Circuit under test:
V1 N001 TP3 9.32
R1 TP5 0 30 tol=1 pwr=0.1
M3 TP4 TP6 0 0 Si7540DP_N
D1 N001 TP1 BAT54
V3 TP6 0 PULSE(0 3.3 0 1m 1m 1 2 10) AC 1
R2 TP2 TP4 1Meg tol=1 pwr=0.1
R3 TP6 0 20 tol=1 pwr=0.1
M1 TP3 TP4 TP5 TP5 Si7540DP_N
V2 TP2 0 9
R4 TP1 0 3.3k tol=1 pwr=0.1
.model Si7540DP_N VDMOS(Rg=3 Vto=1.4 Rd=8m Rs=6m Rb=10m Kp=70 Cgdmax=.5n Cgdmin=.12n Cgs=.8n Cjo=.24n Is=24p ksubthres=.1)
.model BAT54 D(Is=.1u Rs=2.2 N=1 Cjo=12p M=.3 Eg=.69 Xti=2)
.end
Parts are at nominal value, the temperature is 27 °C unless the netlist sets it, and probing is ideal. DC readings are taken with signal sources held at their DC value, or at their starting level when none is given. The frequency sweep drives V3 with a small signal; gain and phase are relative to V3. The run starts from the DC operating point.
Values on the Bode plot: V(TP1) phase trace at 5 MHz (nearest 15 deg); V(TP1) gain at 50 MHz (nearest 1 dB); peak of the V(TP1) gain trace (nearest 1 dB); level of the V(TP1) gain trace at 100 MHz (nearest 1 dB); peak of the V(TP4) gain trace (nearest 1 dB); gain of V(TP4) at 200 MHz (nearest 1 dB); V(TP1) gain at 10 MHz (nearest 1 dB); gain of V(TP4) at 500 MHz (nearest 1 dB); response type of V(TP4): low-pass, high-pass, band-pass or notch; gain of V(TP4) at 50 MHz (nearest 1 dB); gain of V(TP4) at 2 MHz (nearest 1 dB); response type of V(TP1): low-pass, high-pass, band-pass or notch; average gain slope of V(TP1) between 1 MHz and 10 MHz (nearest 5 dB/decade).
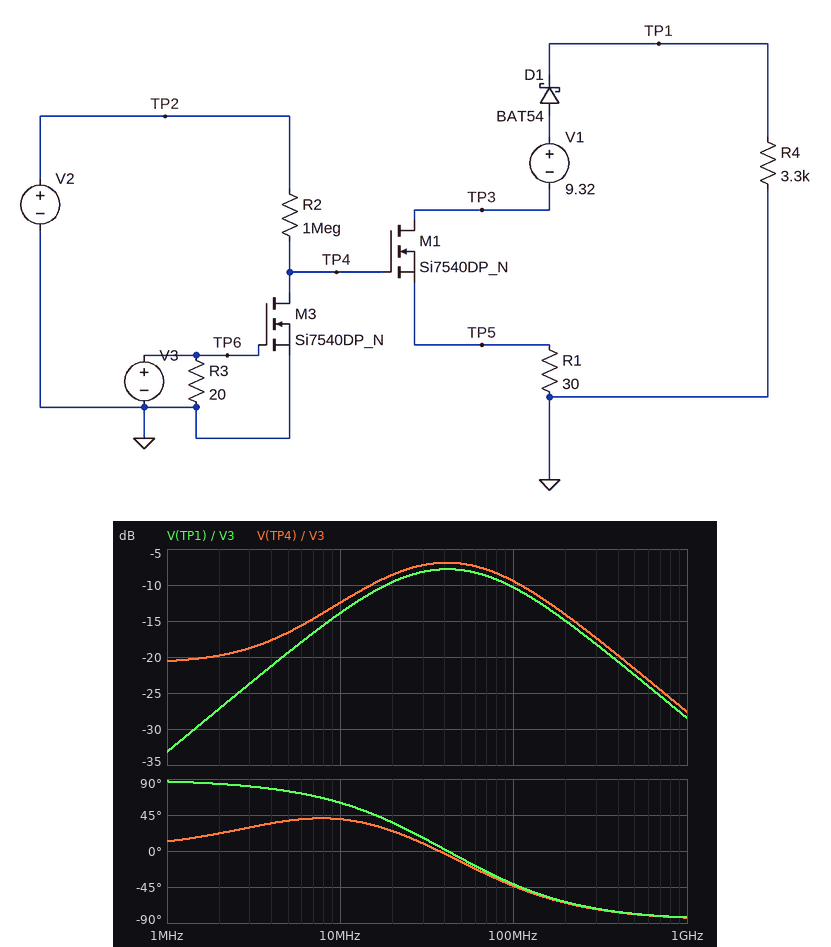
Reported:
75 deg
-8 dB
-8 dB
-10 dB
-7 dB
-14 dB
-14 dB
-22 dB
band-pass
-7 dB
-20 dB
band-pass
20 dB/decade
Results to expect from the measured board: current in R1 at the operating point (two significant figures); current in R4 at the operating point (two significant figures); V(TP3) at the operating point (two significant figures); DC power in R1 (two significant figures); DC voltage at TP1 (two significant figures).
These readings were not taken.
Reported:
2.7 mA
2.7 mA
-82 mV
220 µW
9.0 V
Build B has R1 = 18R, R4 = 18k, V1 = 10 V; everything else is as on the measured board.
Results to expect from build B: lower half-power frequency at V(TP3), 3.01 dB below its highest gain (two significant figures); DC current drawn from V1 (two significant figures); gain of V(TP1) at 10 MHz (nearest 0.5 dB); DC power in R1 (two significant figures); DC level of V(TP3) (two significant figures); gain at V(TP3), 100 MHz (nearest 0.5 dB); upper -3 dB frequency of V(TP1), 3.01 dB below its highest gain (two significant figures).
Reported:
21 MHz
540 µA
-18.0 dB
5.3 µW
-9.8 mV
-11.5 dB
130 MHz
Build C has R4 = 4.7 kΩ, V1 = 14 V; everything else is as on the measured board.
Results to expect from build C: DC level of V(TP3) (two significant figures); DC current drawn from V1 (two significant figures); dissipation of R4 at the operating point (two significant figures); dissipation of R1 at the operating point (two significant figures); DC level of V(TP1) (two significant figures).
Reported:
-87 mV
2.9 mA
40 mW
250 µW
14 V
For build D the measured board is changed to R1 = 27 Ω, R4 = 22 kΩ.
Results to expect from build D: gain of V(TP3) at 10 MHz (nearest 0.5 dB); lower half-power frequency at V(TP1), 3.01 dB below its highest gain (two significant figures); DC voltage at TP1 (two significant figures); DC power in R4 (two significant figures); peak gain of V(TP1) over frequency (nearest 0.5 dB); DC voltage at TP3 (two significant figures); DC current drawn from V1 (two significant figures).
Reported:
-14.5 dB
17 MHz
9.1 V
3.8 mW
-8.0 dB
-11 mV
410 µA
